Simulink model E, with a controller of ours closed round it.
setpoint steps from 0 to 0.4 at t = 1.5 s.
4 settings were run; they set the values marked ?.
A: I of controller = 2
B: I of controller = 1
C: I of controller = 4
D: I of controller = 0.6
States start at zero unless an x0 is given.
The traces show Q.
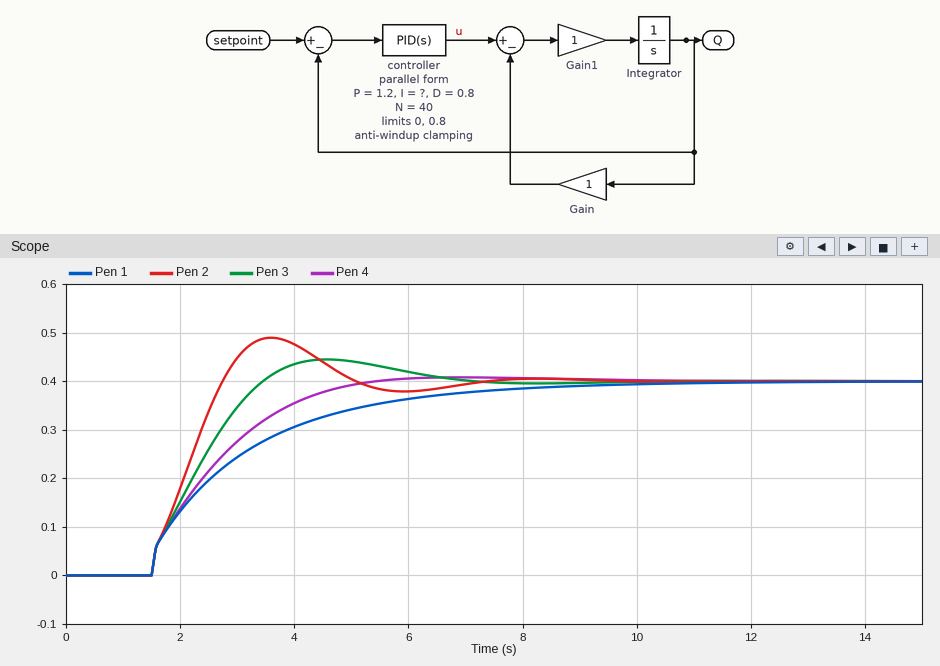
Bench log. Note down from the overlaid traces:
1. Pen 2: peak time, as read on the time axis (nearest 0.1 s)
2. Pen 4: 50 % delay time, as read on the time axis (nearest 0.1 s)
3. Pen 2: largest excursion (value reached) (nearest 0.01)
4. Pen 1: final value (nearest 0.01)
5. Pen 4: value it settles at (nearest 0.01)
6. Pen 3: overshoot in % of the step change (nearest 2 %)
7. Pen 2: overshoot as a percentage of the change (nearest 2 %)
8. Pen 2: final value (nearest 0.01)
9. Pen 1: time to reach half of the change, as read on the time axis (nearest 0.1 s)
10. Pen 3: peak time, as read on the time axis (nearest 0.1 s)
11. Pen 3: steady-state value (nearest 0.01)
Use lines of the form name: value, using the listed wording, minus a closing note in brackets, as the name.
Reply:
Pen 2: peak time, as read on the time axis: 3.6 s
Pen 4: 50 % delay time, as read on the time axis: 2.4 s
Pen 2: largest excursion (value reached): 0.49
Pen 1: final value: 0.40
Pen 4: value it settles at: 0.40
Pen 3: overshoot in % of the step change: 12 %
Pen 2: overshoot as a percentage of the change: 22 %
Pen 2: final value: 0.40
Pen 1: time to reach half of the change, as read on the time axis: 2.5 s
Pen 3: peak time, as read on the time axis: 4.6 s
Pen 3: steady-state value: 0.40
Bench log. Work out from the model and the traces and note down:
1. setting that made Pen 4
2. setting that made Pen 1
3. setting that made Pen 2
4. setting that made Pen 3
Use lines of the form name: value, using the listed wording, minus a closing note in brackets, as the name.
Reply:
setting that made Pen 4: B
setting that made Pen 1: D
setting that made Pen 2: C
setting that made Pen 3: A
